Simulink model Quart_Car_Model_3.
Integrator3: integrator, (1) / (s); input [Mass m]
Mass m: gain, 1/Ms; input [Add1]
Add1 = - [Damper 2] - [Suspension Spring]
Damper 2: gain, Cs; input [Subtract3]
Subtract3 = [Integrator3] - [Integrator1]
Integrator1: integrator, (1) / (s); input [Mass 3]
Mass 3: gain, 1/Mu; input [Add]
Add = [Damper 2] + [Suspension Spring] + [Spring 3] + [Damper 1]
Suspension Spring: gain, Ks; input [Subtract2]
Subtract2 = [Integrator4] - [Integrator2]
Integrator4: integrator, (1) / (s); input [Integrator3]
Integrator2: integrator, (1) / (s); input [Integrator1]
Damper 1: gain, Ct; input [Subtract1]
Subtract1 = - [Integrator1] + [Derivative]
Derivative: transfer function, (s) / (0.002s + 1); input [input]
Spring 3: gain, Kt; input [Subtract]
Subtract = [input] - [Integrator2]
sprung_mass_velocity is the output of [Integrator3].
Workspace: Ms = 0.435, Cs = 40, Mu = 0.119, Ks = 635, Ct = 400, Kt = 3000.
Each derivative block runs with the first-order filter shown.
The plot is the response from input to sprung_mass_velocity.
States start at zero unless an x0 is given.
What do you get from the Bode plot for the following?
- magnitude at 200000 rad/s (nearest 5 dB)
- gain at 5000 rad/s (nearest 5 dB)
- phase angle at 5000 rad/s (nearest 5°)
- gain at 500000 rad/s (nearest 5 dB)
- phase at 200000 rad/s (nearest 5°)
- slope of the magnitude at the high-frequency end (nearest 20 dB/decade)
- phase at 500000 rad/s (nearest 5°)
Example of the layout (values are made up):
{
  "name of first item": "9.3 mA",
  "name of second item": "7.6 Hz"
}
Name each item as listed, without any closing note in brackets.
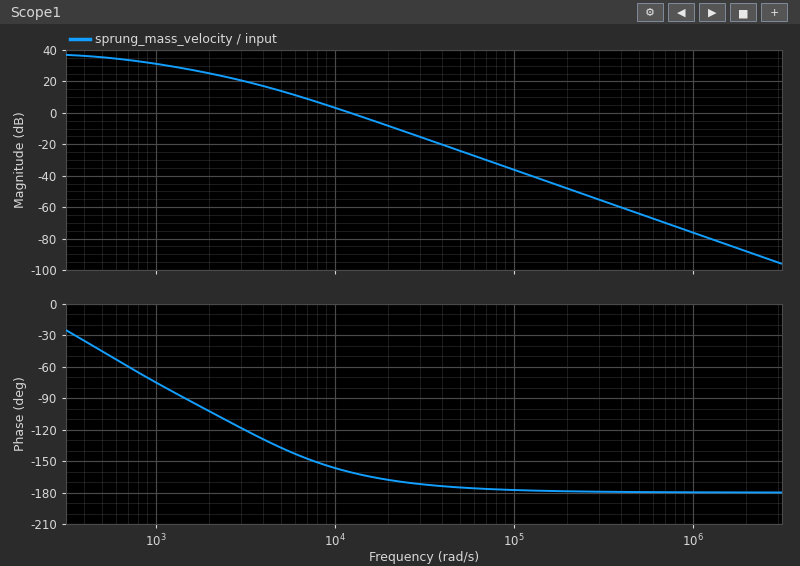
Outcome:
{
  "magnitude at 200000 rad/s": "-50 dB",
  "gain at 5000 rad/s": "15 dB",
  "phase angle at 5000 rad/s": "-135°",
  "gain at 500000 rad/s": "-65 dB",
  "phase at 200000 rad/s": "-180°",
  "slope of the magnitude at the high-frequency end": "-40 dB/decade",
  "phase at 500000 rad/s": "-180°"
}
